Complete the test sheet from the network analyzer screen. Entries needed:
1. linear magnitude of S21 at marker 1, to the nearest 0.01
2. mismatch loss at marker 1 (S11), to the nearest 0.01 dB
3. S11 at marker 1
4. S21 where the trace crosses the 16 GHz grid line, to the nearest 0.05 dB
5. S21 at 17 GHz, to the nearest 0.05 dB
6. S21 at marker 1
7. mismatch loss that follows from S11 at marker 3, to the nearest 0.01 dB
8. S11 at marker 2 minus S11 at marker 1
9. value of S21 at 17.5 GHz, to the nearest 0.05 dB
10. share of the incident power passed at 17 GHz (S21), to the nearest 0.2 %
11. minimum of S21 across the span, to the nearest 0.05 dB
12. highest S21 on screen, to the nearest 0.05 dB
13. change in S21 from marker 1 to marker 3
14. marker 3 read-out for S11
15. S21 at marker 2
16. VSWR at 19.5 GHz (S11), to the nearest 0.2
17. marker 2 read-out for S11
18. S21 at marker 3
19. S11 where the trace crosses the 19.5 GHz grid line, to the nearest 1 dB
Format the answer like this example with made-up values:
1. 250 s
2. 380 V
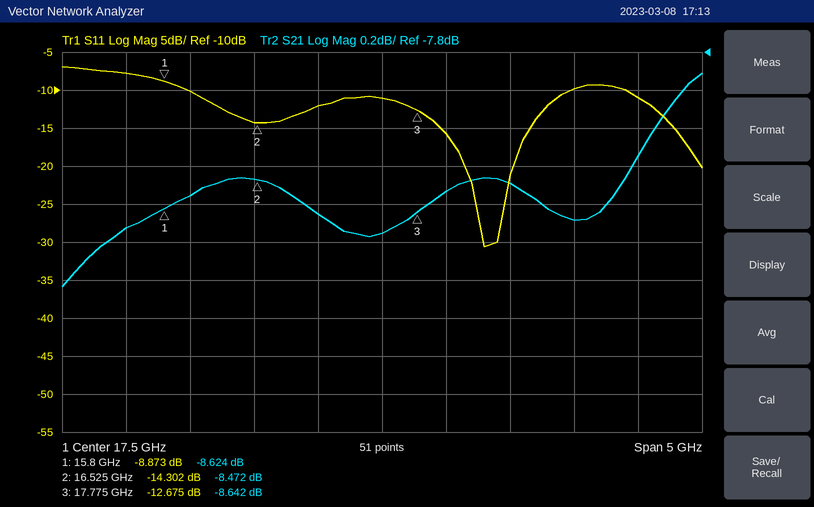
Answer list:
1. 0.37
2. 0.60 dB
3. -8.873 dB
4. -8.55 dB
5. -8.65 dB
6. -8.624 dB
7. 0.24 dB
8. -5.429 dB
9. -8.75 dB
10. 13.6 %
11. -9.05 dB
12. -7.90 dB
13. -0.018 dB
14. -12.675 dB
15. -8.472 dB
16. 1.8
17. -14.302 dB
18. -8.642 dB
19. -11 dB
